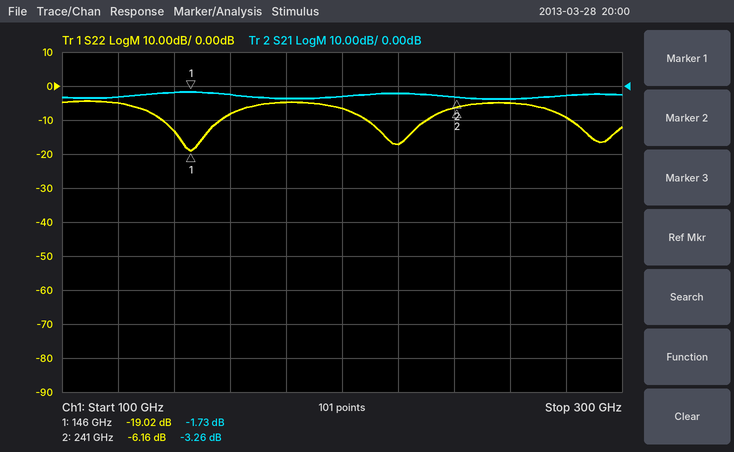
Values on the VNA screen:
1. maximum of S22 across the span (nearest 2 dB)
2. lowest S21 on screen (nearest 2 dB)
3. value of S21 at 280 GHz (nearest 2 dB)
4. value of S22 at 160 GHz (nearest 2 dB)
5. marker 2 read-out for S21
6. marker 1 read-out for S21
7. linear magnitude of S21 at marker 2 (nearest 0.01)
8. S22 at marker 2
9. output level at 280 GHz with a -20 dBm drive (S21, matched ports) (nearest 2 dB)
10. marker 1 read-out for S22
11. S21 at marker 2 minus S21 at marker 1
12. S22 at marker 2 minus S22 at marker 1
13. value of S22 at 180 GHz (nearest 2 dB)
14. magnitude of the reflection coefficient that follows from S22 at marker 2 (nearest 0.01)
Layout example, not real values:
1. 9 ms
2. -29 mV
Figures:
1. -4 dB
2. -4 dB
3. -2 dB
4. -8 dB
5. -3.26 dB
6. -1.73 dB
7. 0.69
8. -6.16 dB
9. -22 dBm
10. -19.02 dB
11. -1.53 dB
12. 12.86 dB
13. -4 dB
14. 0.49
